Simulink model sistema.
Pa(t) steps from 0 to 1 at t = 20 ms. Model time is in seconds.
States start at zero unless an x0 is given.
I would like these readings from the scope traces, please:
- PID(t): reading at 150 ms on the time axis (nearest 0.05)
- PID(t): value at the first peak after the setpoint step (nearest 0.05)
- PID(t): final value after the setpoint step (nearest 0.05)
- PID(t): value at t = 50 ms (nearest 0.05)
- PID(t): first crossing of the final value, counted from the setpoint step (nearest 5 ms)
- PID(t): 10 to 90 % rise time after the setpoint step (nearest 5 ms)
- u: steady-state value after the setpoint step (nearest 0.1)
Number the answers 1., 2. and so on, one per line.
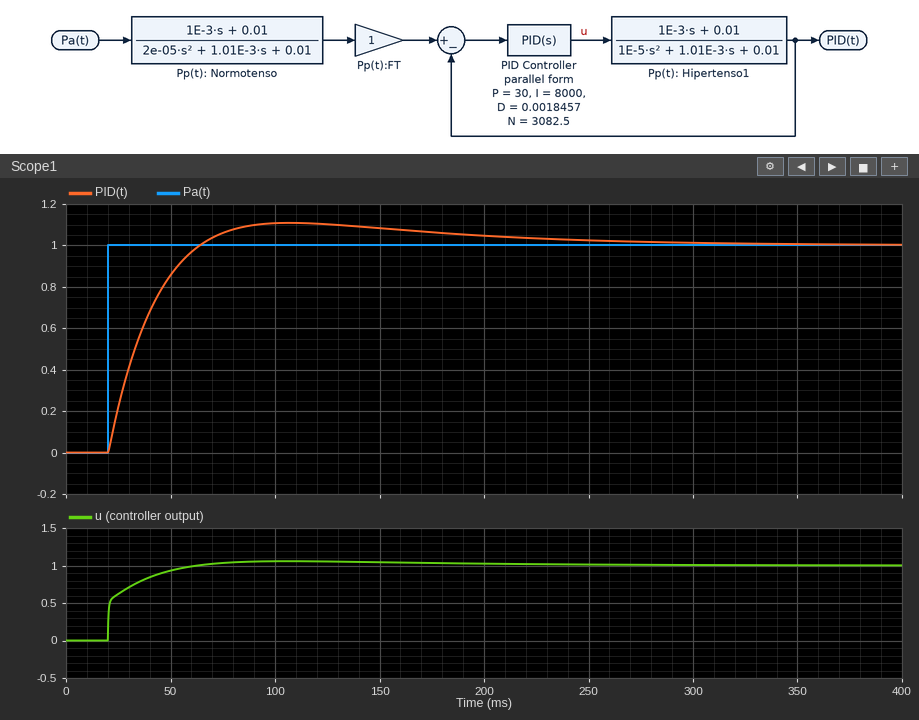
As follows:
1. 1.10
2. 1.10
3. 1.00
4. 0.85
5. 45 ms
6. 30 ms
7. 1.0
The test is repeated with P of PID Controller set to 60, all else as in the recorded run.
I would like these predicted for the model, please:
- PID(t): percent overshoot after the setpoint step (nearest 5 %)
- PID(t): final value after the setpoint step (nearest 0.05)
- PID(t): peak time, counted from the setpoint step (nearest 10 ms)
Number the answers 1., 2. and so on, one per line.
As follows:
1. 10 %
2. 1.00
3. 90 ms
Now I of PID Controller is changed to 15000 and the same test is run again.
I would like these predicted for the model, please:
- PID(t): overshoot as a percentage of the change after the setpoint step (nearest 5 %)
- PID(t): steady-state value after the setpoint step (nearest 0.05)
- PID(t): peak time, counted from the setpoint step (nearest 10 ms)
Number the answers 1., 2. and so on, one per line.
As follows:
1. 10 %
2. 1.00
3. 90 ms
